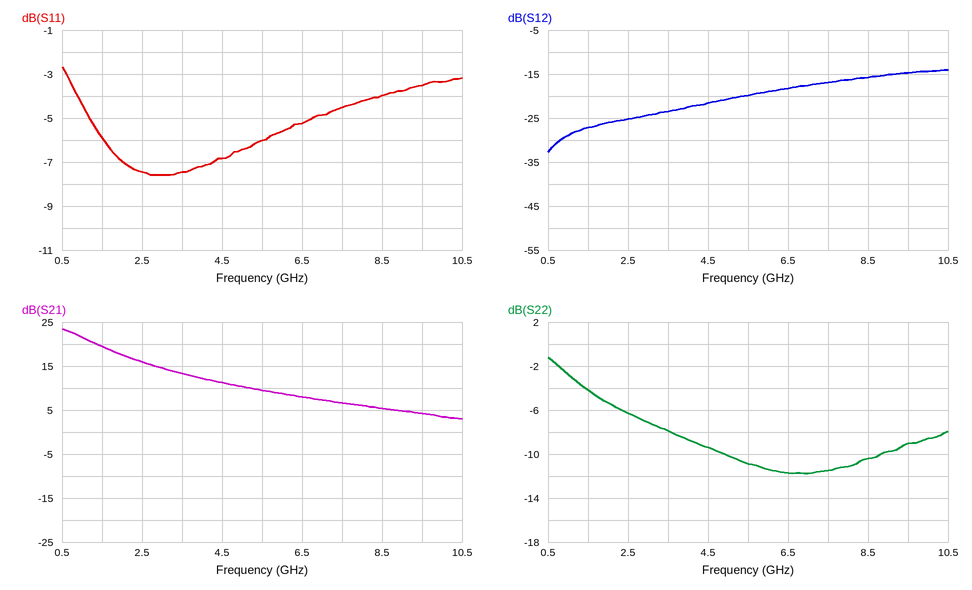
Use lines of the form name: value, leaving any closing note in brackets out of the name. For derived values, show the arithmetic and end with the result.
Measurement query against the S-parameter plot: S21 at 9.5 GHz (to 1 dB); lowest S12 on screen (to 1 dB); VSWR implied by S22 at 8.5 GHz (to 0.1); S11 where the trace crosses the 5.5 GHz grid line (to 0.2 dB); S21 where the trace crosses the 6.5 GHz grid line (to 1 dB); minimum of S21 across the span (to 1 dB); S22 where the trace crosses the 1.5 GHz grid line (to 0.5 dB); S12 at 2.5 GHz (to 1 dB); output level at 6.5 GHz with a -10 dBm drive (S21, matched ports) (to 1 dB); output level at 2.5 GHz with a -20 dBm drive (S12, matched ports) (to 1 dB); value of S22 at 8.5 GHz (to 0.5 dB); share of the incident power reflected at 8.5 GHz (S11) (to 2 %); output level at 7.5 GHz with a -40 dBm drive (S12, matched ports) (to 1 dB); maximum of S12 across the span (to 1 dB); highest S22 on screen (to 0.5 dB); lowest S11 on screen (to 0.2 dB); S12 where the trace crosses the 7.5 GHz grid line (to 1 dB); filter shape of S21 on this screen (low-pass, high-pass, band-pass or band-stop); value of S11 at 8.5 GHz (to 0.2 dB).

S21 at 9.5 GHz: 4 dB
lowest S12 on screen: -33 dB
VSWR implied by S22 at 8.5 GHz: |Γ| = 10^(-10.5/20) = 0.2985; VSWR = (1 + 0.2985)/(1 − 0.2985) ≈ 1.9
S11 where the trace crosses the 5.5 GHz grid line: -6.0 dB
S21 where the trace crosses the 6.5 GHz grid line: 8 dB
minimum of S21 across the span: 3 dB
S22 where the trace crosses the 1.5 GHz grid line: -4.0 dB
S12 at 2.5 GHz: -25 dB
output level at 6.5 GHz with a -10 dBm drive (S21, matched ports): -10 dBm + (8 dB) = -2 dBm
output level at 2.5 GHz with a -20 dBm drive (S12, matched ports): -20 dBm + (-25 dB) = -45 dBm
value of S22 at 8.5 GHz: -10.5 dB
share of the incident power reflected at 8.5 GHz (S11): 10^(-4/10) ≈ 40 %
output level at 7.5 GHz with a -40 dBm drive (S12, matched ports): -40 dBm + (-17 dB) = -57 dBm
maximum of S12 across the span: -14 dB
highest S22 on screen: -1.0 dB
lowest S11 on screen: -7.6 dB
S12 where the trace crosses the 7.5 GHz grid line: -17 dB
filter shape of S21 on this screen: low-pass
value of S11 at 8.5 GHz: -4.0 dB
